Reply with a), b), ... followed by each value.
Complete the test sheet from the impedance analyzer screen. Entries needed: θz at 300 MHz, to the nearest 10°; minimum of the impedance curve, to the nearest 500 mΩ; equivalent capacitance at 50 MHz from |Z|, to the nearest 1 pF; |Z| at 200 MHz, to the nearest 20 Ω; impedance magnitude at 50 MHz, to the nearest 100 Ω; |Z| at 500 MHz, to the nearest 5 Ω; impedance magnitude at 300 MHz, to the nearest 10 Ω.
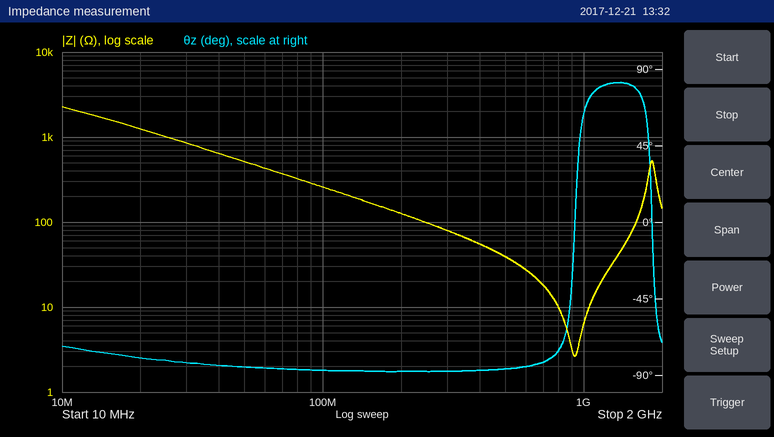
a) -90°
b) 2.5 Ω
c) 6 pF
d) 120 Ω
e) 500 Ω
f) 40 Ω
g) 80 Ω
